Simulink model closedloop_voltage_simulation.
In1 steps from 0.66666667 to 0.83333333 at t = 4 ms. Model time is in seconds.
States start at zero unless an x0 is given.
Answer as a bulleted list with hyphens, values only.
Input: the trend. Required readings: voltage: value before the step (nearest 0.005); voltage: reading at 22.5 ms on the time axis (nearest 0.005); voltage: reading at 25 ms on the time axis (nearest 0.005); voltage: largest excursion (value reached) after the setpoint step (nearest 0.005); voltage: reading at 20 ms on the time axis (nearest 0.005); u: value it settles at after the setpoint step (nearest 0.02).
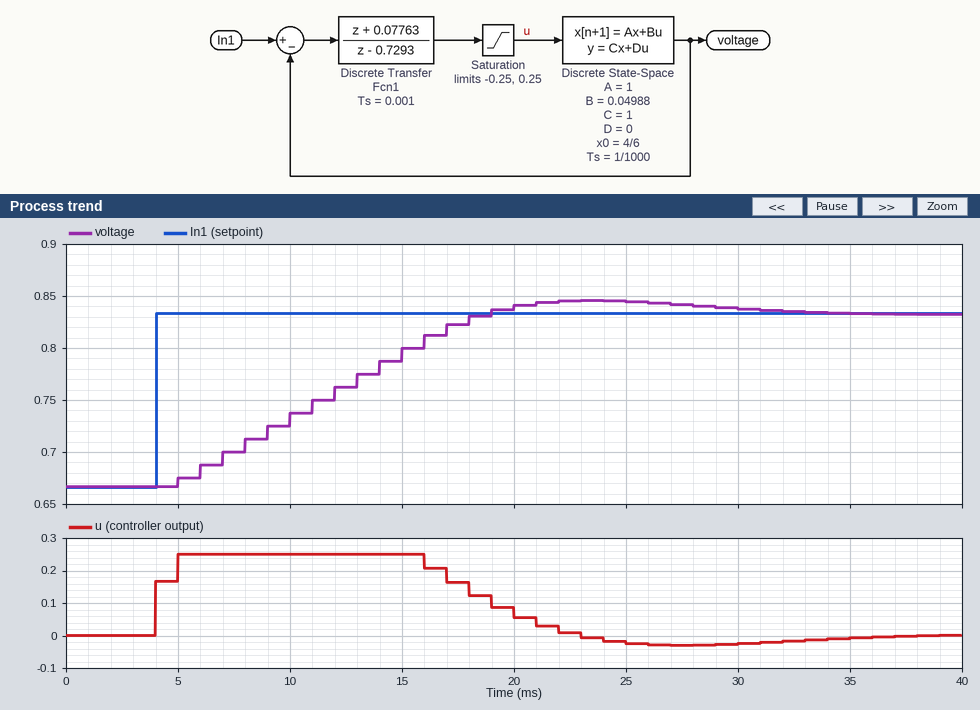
- 0.665
- 0.845
- 0.845
- 0.845
- 0.840
- 0.00
